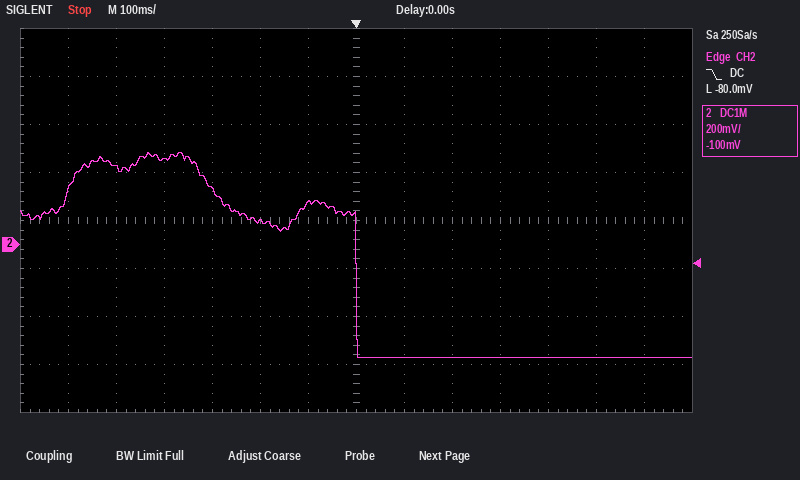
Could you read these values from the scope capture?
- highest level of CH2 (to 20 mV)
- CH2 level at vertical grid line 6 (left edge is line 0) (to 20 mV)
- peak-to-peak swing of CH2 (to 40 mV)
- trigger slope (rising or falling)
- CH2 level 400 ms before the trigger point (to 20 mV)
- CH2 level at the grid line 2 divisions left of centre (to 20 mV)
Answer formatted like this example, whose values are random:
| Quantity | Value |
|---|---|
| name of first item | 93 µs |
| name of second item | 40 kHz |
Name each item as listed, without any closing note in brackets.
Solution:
| Quantity | Value |
|---|---|
| highest level of CH2 | 380 mV |
| CH2 level at vertical grid line 6 (left edge is line 0) | 180 mV |
| peak-to-peak swing of CH2 | 840 mV |
| trigger slope | falling |
| CH2 level 400 ms before the trigger point | 360 mV |
| CH2 level at the grid line 2 divisions left of centre | 100 mV |
